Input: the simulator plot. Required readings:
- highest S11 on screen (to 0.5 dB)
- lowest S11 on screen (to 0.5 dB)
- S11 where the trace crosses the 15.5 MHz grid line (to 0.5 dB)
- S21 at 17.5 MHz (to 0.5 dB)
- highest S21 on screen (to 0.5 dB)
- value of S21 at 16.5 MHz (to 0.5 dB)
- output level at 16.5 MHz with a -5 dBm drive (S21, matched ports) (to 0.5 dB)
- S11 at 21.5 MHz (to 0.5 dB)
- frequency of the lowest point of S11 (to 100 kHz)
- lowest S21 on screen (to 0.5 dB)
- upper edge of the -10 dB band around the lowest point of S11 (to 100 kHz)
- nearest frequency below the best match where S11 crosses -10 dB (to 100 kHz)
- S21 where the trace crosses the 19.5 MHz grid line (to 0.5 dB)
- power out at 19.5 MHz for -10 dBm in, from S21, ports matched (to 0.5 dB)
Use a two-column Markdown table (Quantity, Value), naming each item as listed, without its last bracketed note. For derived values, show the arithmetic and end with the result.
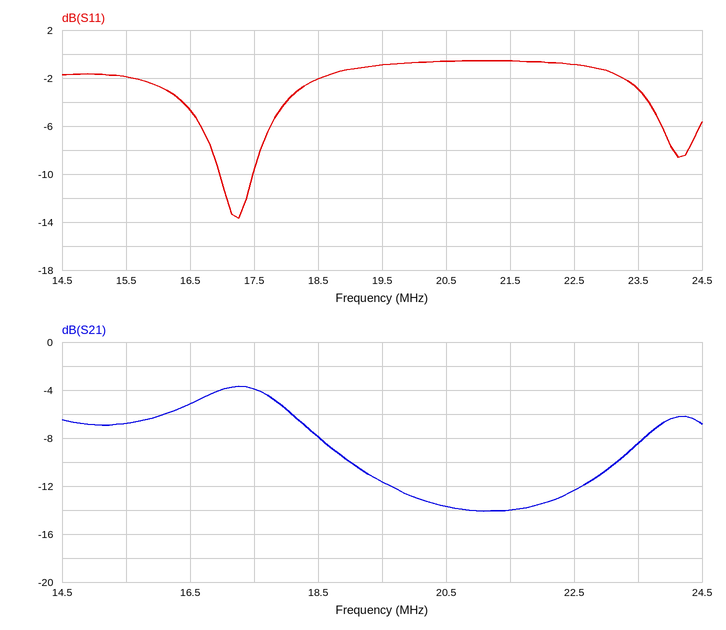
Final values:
| Quantity | Value |
|---|---|
| highest S11 on screen | -0.5 dB |
| lowest S11 on screen | -13.5 dB |
| S11 where the trace crosses the 15.5 MHz grid line | -2.0 dB |
| S21 at 17.5 MHz | -4.0 dB |
| highest S21 on screen | -3.5 dB |
| value of S21 at 16.5 MHz | -5.0 dB |
| output level at 16.5 MHz with a -5 dBm drive (S21, matched ports) | -5 dBm + (-5.0 dB) = -10.0 dBm |
| S11 at 21.5 MHz | -0.5 dB |
| frequency of the lowest point of S11 | 17.3 MHz |
| lowest S21 on screen | -14.0 dB |
| upper edge of the -10 dB band around the lowest point of S11 | 17.5 MHz |
| nearest frequency below the best match where S11 crosses -10 dB | 17.0 MHz |
| S21 where the trace crosses the 19.5 MHz grid line | -11.5 dB |
| power out at 19.5 MHz for -10 dBm in, from S21, ports matched | -10 dBm + (-11.5 dB) = -21.5 dBm |
